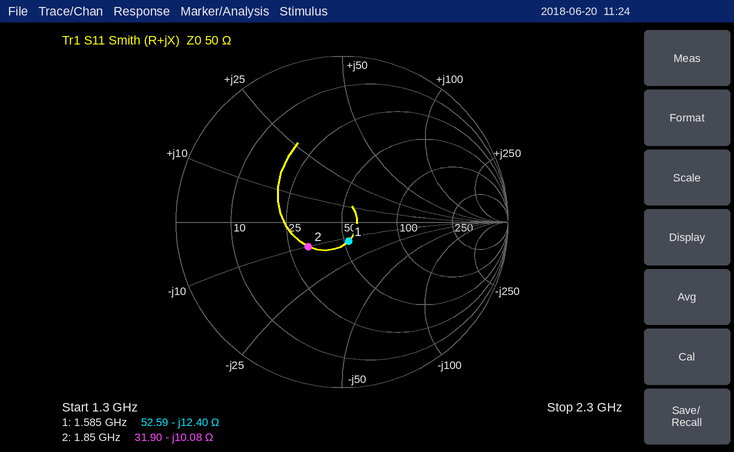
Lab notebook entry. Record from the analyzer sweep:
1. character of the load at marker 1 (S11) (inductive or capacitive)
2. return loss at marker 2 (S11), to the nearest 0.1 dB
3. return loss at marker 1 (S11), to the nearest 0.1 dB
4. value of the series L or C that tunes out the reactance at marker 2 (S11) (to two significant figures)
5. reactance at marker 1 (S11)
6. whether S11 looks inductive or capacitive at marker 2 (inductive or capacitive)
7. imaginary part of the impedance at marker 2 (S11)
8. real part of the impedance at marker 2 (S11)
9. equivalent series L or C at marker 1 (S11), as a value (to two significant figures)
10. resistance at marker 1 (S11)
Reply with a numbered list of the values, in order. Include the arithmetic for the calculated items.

1. capacitive
2. 12.0 dB
3. 18.2 dB
4. L = 10.08 Ω/(2π × 1.85 GHz) ≈ 867 pH, so 870 pH to two significant figures
5. -12.40 Ω
6. capacitive
7. -10.08 Ω
8. 31.90 Ω
9. C = 1/(2π × 1.585 GHz × 12.4 Ω) ≈ 8.1 pF
10. 52.59 Ω
